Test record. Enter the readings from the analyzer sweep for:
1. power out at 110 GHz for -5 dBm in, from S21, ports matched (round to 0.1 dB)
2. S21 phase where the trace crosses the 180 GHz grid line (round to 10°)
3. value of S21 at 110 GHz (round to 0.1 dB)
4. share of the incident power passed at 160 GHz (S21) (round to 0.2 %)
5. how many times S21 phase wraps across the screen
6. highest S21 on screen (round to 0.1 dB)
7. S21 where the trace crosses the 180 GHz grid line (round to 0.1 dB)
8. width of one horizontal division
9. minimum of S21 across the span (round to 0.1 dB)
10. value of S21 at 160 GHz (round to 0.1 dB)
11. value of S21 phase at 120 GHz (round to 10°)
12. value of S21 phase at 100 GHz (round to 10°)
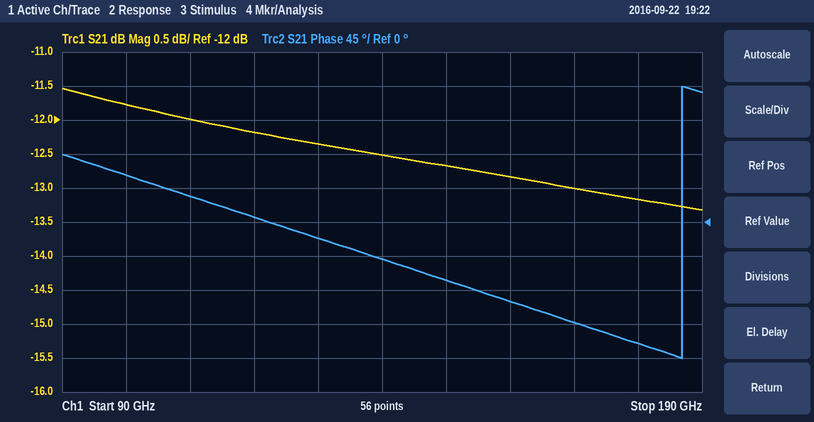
-17.0 dBm
-160°
-12.0 dB
5.2 %
1
-11.5 dB
-13.2 dB
10 GHz
-13.3 dB
-12.8 dB
10°
60°
